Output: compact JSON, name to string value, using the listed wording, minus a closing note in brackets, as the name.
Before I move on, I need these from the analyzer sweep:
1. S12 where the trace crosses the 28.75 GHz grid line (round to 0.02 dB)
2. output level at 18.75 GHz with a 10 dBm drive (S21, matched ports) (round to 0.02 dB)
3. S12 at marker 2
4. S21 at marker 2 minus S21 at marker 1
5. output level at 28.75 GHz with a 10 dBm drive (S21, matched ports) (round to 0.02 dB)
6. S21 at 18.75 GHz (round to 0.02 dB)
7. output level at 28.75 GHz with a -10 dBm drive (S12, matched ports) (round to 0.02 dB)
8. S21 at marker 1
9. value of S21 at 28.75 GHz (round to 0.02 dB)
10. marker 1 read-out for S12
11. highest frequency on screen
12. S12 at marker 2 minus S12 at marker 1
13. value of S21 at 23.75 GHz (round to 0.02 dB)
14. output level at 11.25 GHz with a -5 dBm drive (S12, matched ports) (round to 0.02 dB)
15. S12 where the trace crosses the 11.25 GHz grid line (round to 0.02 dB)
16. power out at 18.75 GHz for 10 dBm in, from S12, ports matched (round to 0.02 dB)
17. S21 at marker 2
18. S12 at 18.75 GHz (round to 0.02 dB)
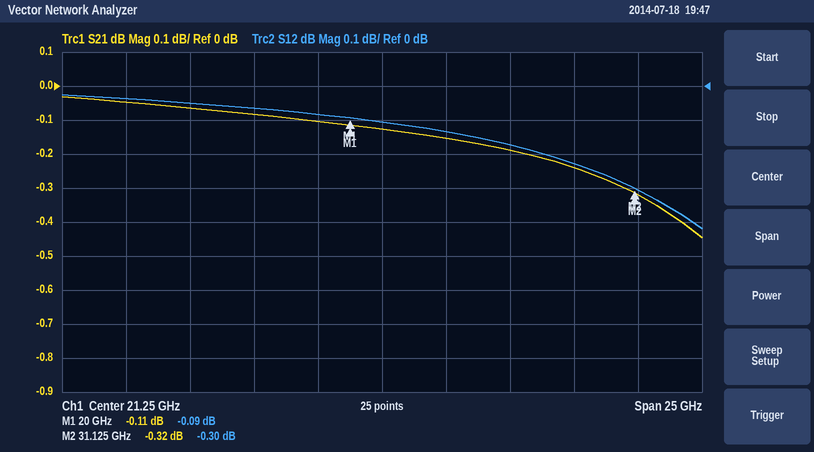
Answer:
{"S12 where the trace crosses the 28.75 GHz grid line": "-0.22 dB", "output level at 18.75 GHz with a 10 dBm drive (S21, matched ports)": "9.90 dBm", "S12 at marker 2": "-0.30 dB", "S21 at marker 2 minus S21 at marker 1": "-0.21 dB", "output level at 28.75 GHz with a 10 dBm drive (S21, matched ports)": "9.76 dBm", "S21 at 18.75 GHz": "-0.10 dB", "output level at 28.75 GHz with a -10 dBm drive (S12, matched ports)": "-10.22 dBm", "S21 at marker 1": "-0.11 dB", "value of S21 at 28.75 GHz": "-0.24 dB", "marker 1 read-out for S12": "-0.09 dB", "highest frequency on screen": "33.75 GHz", "S12 at marker 2 minus S12 at marker 1": "-0.21 dB", "value of S21 at 23.75 GHz": "-0.16 dB", "output level at 11.25 GHz with a -5 dBm drive (S12, matched ports)": "-5.04 dBm", "S12 where the trace crosses the 11.25 GHz grid line": "-0.04 dB", "power out at 18.75 GHz for 10 dBm in, from S12, ports matched": "9.92 dBm", "S21 at marker 2": "-0.32 dB", "S12 at 18.75 GHz": "-0.08 dB"}
